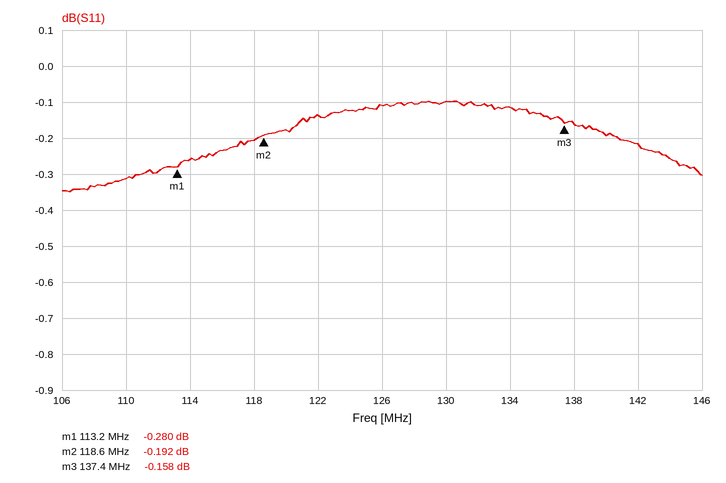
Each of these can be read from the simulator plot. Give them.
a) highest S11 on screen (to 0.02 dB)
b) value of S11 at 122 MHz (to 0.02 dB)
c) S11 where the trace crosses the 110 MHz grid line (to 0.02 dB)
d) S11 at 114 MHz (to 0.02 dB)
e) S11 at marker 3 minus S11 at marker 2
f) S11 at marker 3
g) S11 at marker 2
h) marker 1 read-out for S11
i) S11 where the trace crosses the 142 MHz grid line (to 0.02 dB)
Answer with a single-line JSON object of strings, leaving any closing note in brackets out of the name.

{"highest S11 on screen": "-0.10 dB", "value of S11 at 122 MHz": "-0.14 dB", "S11 where the trace crosses the 110 MHz grid line": "-0.32 dB", "S11 at 114 MHz": "-0.26 dB", "S11 at marker 3 minus S11 at marker 2": "0.034 dB", "S11 at marker 3": "-0.158 dB", "S11 at marker 2": "-0.192 dB", "marker 1 read-out for S11": "-0.280 dB", "S11 where the trace crosses the 142 MHz grid line": "-0.22 dB"}
